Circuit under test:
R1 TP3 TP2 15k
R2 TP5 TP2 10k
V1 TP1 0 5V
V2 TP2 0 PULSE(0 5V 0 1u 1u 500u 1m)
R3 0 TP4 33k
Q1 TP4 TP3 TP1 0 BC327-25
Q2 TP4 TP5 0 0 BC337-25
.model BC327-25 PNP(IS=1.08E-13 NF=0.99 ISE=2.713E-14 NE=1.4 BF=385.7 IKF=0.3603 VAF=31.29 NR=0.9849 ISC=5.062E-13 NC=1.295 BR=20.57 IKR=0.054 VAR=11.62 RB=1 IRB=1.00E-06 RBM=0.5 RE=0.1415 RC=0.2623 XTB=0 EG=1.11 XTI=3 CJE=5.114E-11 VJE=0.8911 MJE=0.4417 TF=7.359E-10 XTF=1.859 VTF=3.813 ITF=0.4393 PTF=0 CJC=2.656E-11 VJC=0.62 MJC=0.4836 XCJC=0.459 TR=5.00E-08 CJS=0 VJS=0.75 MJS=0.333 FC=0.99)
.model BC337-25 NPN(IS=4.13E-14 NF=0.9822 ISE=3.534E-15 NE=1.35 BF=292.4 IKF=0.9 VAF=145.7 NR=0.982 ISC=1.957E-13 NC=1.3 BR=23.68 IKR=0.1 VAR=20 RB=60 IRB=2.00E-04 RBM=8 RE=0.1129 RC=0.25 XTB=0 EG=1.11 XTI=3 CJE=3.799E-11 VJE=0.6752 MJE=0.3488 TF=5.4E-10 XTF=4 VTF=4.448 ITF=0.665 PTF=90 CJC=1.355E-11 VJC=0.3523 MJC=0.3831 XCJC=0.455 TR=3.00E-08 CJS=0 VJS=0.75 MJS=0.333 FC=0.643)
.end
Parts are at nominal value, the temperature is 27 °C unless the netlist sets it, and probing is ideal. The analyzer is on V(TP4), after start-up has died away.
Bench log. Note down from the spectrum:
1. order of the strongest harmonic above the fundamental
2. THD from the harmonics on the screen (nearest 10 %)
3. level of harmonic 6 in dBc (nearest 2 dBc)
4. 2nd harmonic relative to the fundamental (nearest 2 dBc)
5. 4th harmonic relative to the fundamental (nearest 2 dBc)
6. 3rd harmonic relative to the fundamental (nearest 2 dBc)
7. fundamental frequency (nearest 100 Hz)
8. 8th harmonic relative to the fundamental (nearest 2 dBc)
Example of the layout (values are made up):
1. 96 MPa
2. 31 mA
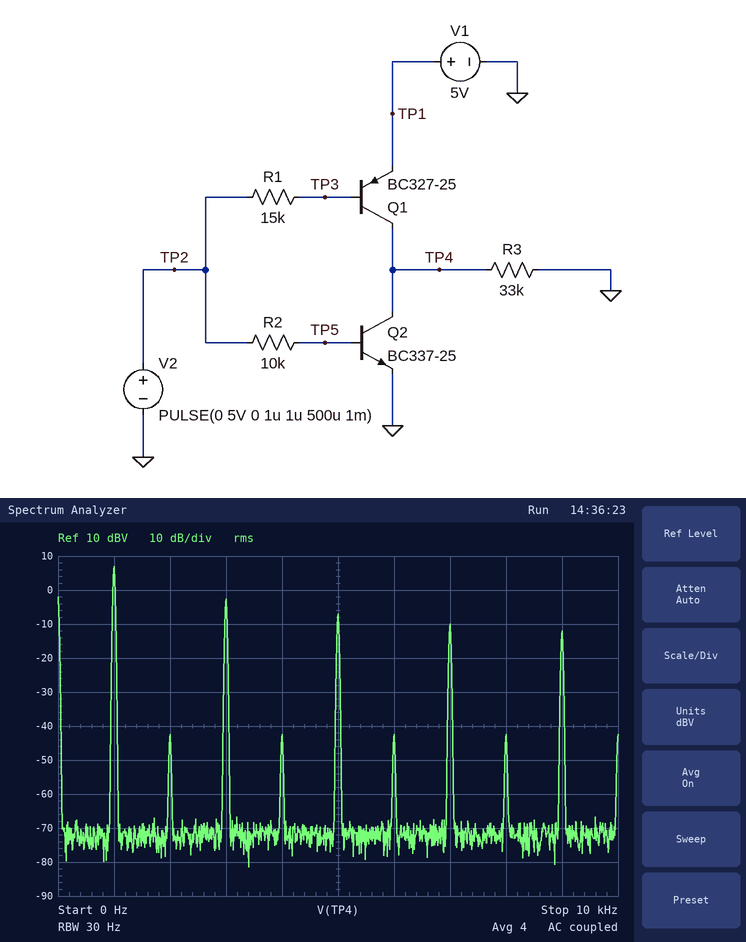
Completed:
1. 3
2. 40 %
3. -50 dBc
4. -50 dBc
5. -50 dBc
6. -10 dBc
7. 1.0 kHz
8. -50 dBc
